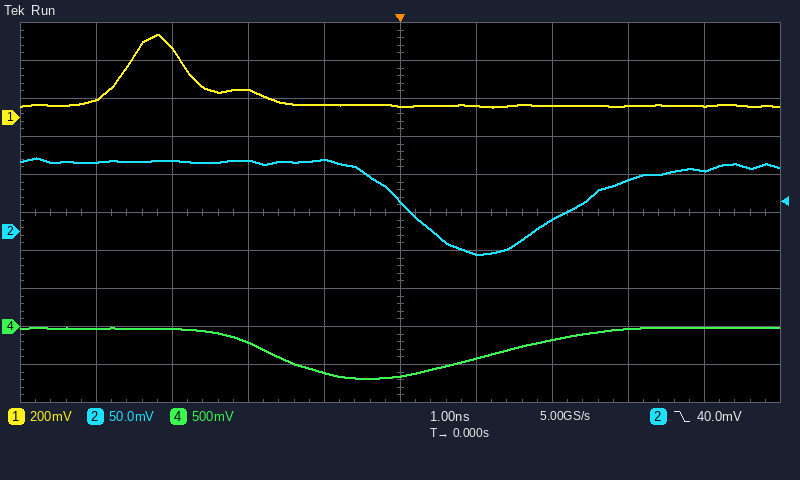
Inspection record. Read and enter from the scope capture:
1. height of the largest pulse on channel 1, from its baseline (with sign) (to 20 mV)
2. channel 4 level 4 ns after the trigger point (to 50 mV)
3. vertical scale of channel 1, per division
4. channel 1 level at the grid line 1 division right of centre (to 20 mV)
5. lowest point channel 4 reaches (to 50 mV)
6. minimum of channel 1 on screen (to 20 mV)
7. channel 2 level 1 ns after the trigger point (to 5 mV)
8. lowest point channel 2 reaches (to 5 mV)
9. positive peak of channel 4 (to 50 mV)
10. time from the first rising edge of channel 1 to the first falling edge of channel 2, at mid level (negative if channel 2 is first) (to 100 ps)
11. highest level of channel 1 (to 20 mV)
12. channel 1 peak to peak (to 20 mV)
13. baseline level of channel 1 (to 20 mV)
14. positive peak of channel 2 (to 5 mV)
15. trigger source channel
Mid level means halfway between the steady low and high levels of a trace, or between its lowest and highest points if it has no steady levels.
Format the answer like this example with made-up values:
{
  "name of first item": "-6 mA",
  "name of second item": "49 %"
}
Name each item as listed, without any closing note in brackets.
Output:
{
  "height of the largest pulse on channel 1, from its baseline (with sign)": "+380 mV",
  "channel 4 level 4 ns after the trigger point": "0 mV",
  "vertical scale of channel 1, per division": "200 mV",
  "channel 1 level at the grid line 1 division right of centre": "60 mV",
  "lowest point channel 4 reaches": "-700 mV",
  "minimum of channel 1 on screen": "60 mV",
  "channel 2 level 1 ns after the trigger point": "-30 mV",
  "lowest point channel 2 reaches": "-30 mV",
  "positive peak of channel 4": "0 mV",
  "time from the first rising edge of channel 1 to the first falling edge of channel 2, at mid level (negative if channel 2 is first)": "+3.7 ns",
  "highest level of channel 1": "440 mV",
  "channel 1 peak to peak": "380 mV",
  "baseline level of channel 1": "60 mV",
  "positive peak of channel 2": "95 mV",
  "trigger source channel": "channel 2"
}
